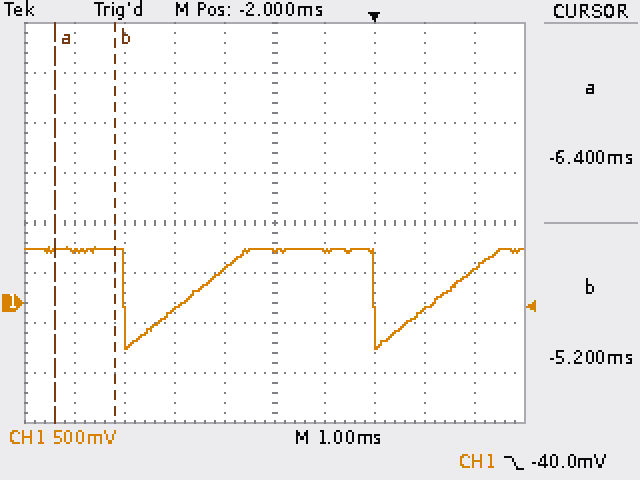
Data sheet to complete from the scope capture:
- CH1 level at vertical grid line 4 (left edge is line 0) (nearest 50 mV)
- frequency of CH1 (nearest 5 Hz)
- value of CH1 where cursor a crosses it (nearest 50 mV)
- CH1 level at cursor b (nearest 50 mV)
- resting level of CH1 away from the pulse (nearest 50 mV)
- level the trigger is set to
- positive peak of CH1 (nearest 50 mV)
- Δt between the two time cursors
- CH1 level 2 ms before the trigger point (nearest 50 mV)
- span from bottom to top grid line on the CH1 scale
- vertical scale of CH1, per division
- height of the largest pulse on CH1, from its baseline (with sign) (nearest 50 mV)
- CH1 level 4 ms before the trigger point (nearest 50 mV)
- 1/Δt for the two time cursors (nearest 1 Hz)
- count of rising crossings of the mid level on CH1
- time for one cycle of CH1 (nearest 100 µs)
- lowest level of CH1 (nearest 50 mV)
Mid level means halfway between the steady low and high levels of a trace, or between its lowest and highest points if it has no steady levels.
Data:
350 mV
200 Hz
550 mV
550 mV
550 mV
-40.0 mV
550 mV
1.2 ms
500 mV
4 V
500 mV
-1.00 V
-50 mV
833 Hz
2
5.0 ms
-450 mV
